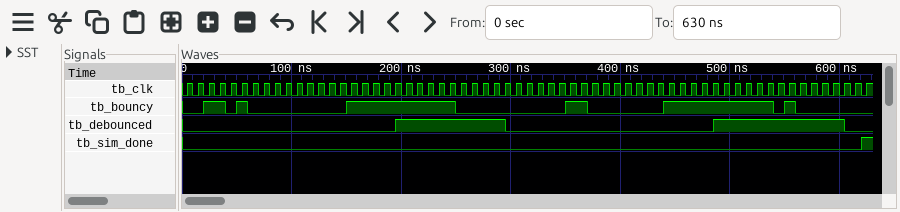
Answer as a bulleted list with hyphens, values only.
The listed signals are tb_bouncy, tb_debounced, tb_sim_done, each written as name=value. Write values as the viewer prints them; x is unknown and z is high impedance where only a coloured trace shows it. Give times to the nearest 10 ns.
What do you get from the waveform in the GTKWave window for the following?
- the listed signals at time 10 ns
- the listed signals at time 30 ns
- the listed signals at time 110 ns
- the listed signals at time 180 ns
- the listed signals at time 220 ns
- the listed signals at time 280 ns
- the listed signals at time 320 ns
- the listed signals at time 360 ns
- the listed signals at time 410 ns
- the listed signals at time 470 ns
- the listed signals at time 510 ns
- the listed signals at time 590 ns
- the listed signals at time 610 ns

- tb_bouncy=0, tb_debounced=0, tb_sim_done=0
- tb_bouncy=1, tb_debounced=0, tb_sim_done=0
- tb_bouncy=0, tb_debounced=0, tb_sim_done=0
- tb_bouncy=1, tb_debounced=0, tb_sim_done=0
- tb_bouncy=1, tb_debounced=1, tb_sim_done=0
- tb_bouncy=0, tb_debounced=1, tb_sim_done=0
- tb_bouncy=0, tb_debounced=0, tb_sim_done=0
- tb_bouncy=1, tb_debounced=0, tb_sim_done=0
- tb_bouncy=0, tb_debounced=0, tb_sim_done=0
- tb_bouncy=1, tb_debounced=0, tb_sim_done=0
- tb_bouncy=1, tb_debounced=1, tb_sim_done=0
- tb_bouncy=0, tb_debounced=1, tb_sim_done=0
- tb_bouncy=0, tb_debounced=0, tb_sim_done=0
